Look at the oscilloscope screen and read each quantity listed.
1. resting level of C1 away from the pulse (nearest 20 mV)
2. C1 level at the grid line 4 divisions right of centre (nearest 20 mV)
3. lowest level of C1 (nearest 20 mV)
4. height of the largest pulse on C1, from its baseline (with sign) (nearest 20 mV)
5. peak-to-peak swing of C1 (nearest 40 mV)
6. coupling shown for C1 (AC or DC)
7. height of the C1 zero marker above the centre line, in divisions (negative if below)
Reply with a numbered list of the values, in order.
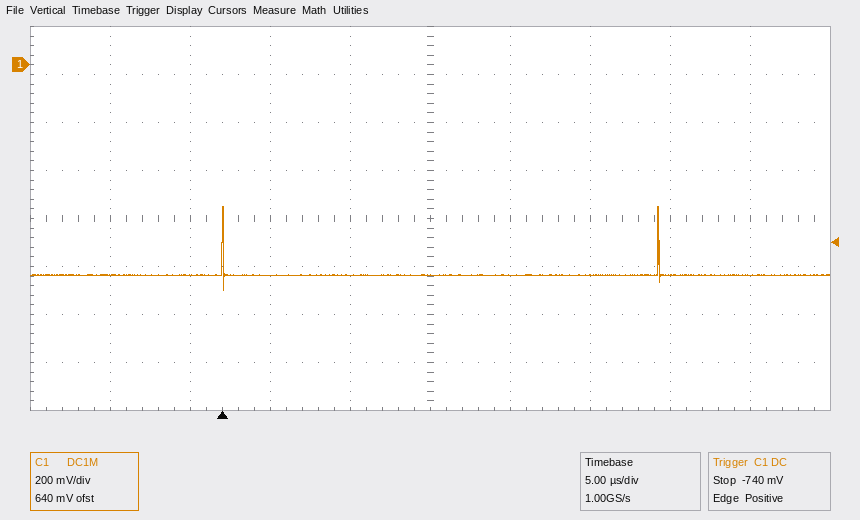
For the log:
1. -880 mV
2. -880 mV
3. -940 mV
4. +280 mV
5. 360 mV
6. DC
7. +3.2 div
